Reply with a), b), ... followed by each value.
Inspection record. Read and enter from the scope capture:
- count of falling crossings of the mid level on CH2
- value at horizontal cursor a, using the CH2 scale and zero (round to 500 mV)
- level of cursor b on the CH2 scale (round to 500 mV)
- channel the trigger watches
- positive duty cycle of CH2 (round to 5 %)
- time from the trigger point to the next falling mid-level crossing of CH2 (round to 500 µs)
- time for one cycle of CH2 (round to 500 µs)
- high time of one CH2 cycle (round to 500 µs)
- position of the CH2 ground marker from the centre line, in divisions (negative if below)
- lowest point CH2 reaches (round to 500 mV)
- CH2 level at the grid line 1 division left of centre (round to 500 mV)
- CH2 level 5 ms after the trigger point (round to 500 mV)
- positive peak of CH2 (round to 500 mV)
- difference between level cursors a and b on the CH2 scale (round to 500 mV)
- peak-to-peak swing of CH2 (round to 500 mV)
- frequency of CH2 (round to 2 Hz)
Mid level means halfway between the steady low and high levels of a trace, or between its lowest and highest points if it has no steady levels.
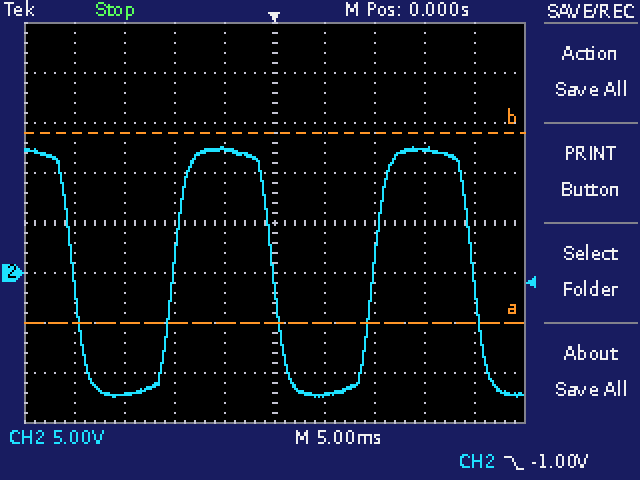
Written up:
a) 3
b) -5.0 V
c) 14.0 V
d) CH2
e) 50 %
f) 20.0 ms
g) 20.0 ms
h) 10.0 ms
i) -1.0 div
j) -12.5 V
k) 12.5 V
l) -12.0 V
m) 12.5 V
n) 19.0 V
o) 25.0 V
p) 50 Hz
